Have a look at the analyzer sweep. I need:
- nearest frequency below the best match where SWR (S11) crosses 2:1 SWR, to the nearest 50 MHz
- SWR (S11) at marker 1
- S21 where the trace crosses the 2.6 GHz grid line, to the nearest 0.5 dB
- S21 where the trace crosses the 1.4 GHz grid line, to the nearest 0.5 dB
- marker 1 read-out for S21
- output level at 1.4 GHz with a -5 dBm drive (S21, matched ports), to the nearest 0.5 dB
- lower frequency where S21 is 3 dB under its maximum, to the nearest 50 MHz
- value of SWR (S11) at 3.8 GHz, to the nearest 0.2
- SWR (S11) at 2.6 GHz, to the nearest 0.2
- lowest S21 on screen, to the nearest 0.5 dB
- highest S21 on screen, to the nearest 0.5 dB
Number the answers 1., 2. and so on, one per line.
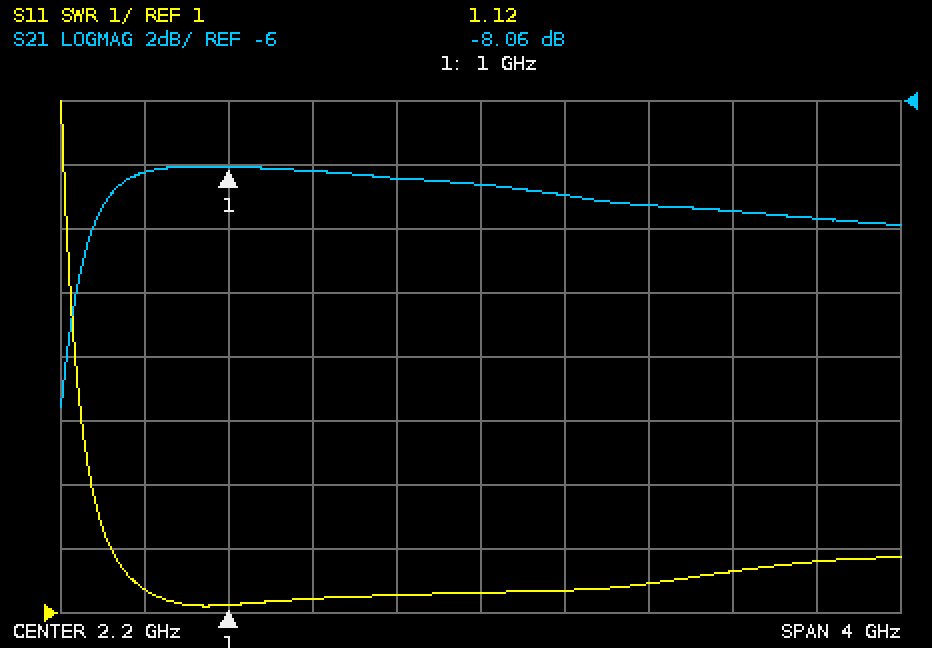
1. 450 MHz
2. 1.12
3. -9.0 dB
4. -8.0 dB
5. -8.06 dB
6. -13.0 dBm
7. 300 MHz
8. 1.8
9. 1.4
10. -15.5 dB
11. -8.0 dB
